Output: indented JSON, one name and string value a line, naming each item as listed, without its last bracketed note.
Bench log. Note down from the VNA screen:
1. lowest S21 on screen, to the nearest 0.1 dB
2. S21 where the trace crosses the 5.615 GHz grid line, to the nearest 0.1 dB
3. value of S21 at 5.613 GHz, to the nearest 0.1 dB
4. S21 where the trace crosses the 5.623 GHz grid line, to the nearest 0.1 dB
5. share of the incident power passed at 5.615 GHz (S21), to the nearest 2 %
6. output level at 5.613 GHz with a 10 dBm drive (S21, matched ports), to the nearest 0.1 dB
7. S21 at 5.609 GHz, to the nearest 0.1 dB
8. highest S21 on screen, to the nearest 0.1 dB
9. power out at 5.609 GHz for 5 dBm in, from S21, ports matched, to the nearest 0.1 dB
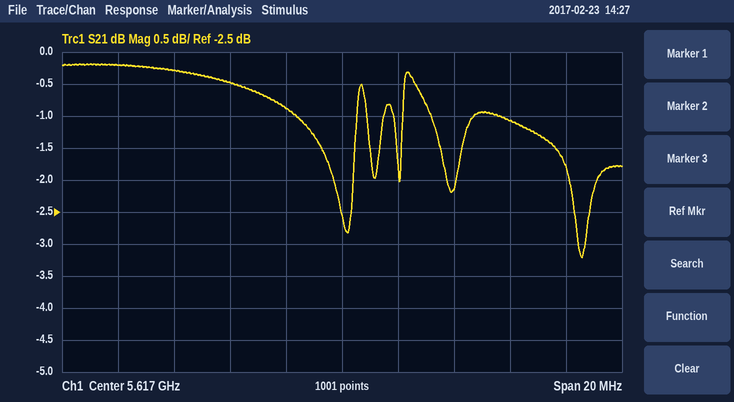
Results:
{
  "lowest S21 on screen, to the nearest 0.1 dB": "-3.2 dB",
  "S21 where the trace crosses the 5.615 GHz grid line, to the nearest 0.1 dB": "-0.9 dB",
  "value of S21 at 5.613 GHz, to the nearest 0.1 dB": "-0.5 dB",
  "S21 where the trace crosses the 5.623 GHz grid line, to the nearest 0.1 dB": "-1.1 dB",
  "share of the incident power passed at 5.615 GHz (S21), to the nearest 2 %": "82 %",
  "output level at 5.613 GHz with a 10 dBm drive (S21, matched ports), to the nearest 0.1 dB": "9.5 dBm",
  "S21 at 5.609 GHz, to the nearest 0.1 dB": "-0.2 dB",
  "highest S21 on screen, to the nearest 0.1 dB": "-0.2 dB",
  "power out at 5.609 GHz for 5 dBm in, from S21, ports matched, to the nearest 0.1 dB": "4.8 dBm"
}
